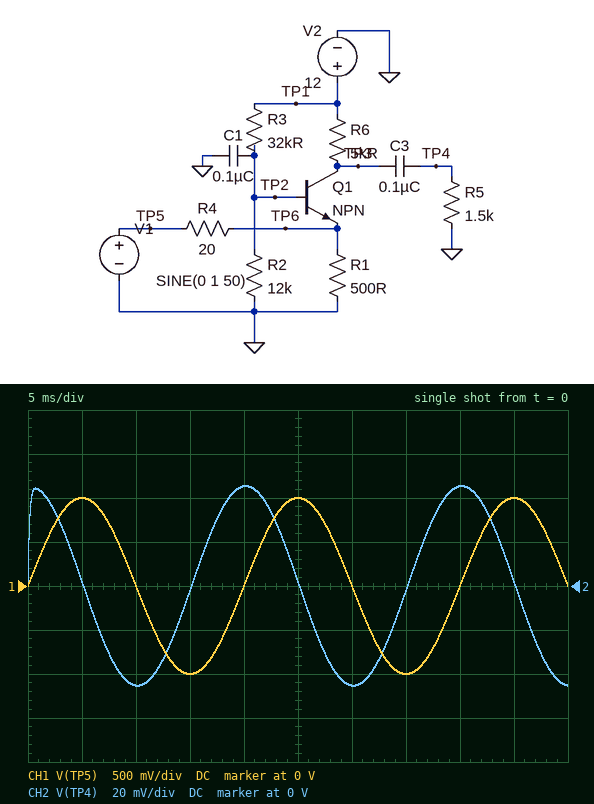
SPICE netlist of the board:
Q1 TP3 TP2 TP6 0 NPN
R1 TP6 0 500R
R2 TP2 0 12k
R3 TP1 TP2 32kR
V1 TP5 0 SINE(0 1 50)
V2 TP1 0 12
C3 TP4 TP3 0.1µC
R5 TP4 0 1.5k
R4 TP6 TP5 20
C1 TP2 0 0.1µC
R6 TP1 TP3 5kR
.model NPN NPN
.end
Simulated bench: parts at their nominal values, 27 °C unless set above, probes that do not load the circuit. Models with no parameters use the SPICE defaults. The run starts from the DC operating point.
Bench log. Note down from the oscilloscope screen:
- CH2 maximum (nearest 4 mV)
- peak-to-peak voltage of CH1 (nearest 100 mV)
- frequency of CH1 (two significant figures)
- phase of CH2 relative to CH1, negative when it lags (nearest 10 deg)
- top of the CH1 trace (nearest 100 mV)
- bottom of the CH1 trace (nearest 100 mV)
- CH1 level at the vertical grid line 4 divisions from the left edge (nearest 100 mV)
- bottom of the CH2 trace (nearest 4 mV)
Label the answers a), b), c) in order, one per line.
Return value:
a) 44 mV
b) 2.0 V
c) 50 Hz
d) 90 deg
e) 1.0 V
f) -1.0 V
g) 0 V
h) -44 mV
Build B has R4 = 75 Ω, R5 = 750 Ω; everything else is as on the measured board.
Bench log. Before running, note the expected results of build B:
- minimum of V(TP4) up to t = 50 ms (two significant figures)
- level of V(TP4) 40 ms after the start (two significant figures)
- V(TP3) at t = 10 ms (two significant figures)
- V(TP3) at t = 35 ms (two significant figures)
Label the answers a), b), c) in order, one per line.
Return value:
a) -20 mV
b) 20 mV
c) 240 mV
d) -620 mV
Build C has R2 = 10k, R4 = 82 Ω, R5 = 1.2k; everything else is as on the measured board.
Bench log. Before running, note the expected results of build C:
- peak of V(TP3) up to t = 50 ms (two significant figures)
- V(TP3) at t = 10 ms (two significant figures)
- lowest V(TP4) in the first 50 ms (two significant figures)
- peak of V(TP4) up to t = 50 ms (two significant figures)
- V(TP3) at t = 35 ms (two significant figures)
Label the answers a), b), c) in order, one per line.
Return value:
a) 1.1 V
b) 250 mV
c) -32 mV
d) 32 mV
e) -600 mV
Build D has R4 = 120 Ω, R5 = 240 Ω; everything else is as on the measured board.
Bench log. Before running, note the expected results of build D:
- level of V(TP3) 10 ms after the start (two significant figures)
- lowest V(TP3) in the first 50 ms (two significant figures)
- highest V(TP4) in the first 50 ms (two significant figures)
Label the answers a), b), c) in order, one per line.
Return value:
a) 320 mV
b) -470 mV
c) 6.0 mV
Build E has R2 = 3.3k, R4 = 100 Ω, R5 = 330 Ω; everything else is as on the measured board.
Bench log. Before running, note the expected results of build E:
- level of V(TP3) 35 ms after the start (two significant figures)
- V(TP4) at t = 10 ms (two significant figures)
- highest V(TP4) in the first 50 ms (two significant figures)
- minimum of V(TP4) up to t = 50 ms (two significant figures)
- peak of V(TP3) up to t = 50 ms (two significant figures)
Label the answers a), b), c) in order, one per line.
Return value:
a) -540 mV
b) -320 mV
c) 240 mV
d) -330 mV
e) 12 V
